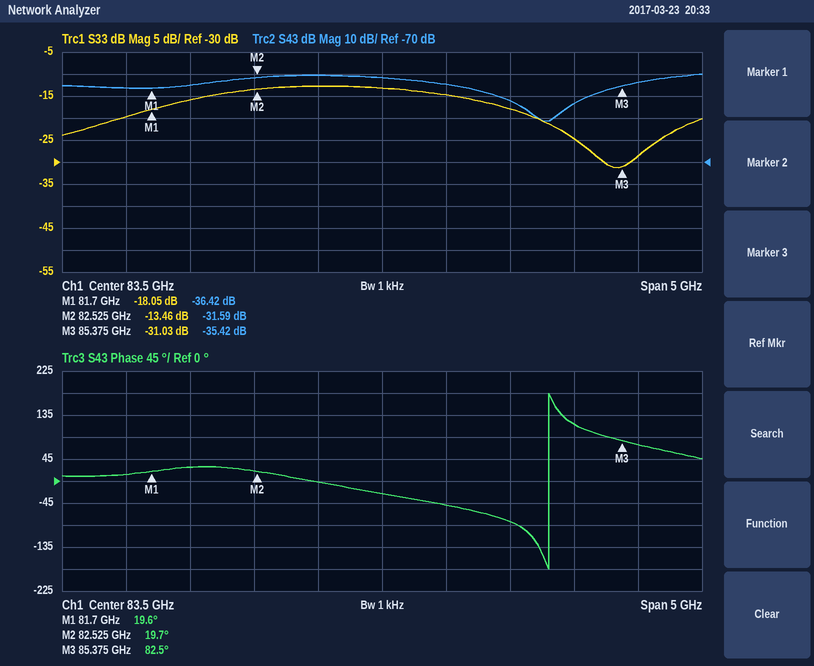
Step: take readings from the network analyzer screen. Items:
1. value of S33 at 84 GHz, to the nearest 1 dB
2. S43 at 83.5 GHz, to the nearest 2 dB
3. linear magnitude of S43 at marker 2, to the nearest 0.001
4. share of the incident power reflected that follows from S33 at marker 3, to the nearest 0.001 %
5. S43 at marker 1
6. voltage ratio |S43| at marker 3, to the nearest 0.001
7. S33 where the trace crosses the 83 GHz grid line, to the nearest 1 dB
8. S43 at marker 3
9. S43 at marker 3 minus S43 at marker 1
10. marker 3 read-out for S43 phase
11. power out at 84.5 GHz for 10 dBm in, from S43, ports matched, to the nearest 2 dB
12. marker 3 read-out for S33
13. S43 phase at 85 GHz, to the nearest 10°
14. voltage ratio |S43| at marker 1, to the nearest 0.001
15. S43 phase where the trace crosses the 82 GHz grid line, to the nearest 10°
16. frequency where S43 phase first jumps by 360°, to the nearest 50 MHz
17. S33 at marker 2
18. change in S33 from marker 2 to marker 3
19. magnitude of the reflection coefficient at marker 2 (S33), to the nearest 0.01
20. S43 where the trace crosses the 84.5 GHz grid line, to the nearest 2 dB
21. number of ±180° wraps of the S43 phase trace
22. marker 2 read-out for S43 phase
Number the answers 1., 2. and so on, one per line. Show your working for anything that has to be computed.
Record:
1. -15 dB
2. -32 dB
3. 10^(-31.59/20) ≈ 0.026
4. 10^(-31.03/10) ≈ 0.079 %
5. -36.42 dB
6. 10^(-35.42/20) ≈ 0.017
7. -13 dB
8. -35.42 dB
9. -35.42 − (-36.42) = 1.00 dB
10. 82.5°
11. 10 dBm + (-42 dB) = -32 dBm
12. -31.03 dB
13. 120°
14. 10^(-36.42/20) ≈ 0.015
15. 30°
16. 84.80 GHz
17. -13.46 dB
18. -31.03 − (-13.46) = -17.57 dB
19. 10^(-13.46/20) ≈ 0.21
20. -42 dB
21. 1
22. 19.7°
